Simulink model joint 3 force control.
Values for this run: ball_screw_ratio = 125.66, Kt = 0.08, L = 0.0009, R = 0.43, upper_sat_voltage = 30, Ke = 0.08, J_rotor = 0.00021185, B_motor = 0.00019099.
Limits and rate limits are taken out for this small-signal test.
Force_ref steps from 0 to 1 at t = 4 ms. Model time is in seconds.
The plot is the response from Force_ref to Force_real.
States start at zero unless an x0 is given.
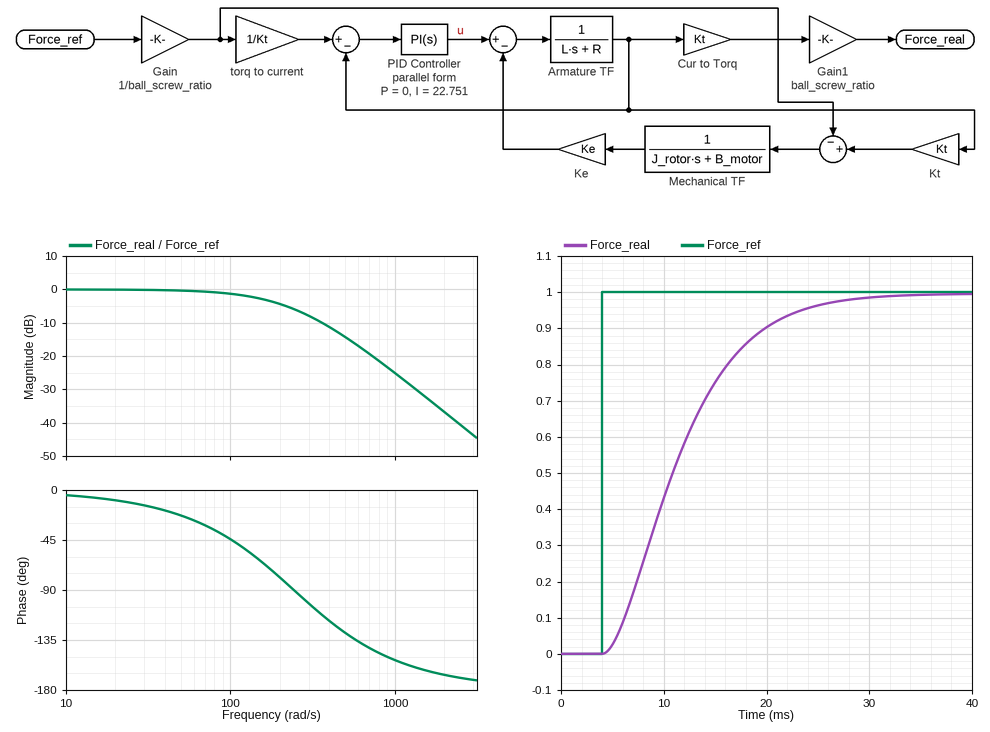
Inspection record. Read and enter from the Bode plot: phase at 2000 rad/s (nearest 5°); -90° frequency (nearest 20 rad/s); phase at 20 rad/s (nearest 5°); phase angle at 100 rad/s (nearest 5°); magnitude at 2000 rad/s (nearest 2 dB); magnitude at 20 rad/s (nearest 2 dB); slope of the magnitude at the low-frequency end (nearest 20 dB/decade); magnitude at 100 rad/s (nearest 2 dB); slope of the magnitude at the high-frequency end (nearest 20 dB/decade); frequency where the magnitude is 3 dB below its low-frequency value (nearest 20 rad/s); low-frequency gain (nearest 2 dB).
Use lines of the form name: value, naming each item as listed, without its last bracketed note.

phase at 2000 rad/s: -165°
-90° frequency: 240 rad/s
phase at 20 rad/s: -10°
phase angle at 100 rad/s: -45°
magnitude at 2000 rad/s: -36 dB
magnitude at 20 rad/s: 0 dB
slope of the magnitude at the low-frequency end: 0 dB/decade
magnitude at 100 rad/s: -2 dB
slope of the magnitude at the high-frequency end: -40 dB/decade
frequency where the magnitude is 3 dB below its low-frequency value: 160 rad/s
low-frequency gain: 0 dB
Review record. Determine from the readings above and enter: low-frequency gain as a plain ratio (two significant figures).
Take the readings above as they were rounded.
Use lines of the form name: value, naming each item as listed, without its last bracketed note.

low-frequency gain as a plain ratio: 1.0
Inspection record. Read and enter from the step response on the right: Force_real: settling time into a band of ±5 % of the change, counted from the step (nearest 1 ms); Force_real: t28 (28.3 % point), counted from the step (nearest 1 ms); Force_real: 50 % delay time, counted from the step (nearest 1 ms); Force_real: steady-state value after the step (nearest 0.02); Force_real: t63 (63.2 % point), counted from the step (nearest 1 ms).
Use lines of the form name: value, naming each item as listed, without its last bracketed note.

Force_real: settling time into a band of ±5 % of the change, counted from the step: 19 ms
Force_real: t28 (28.3 % point), counted from the step: 4 ms
Force_real: 50 % delay time, counted from the step: 7 ms
Force_real: steady-state value after the step: 1.00
Force_real: t63 (63.2 % point), counted from the step: 9 ms
